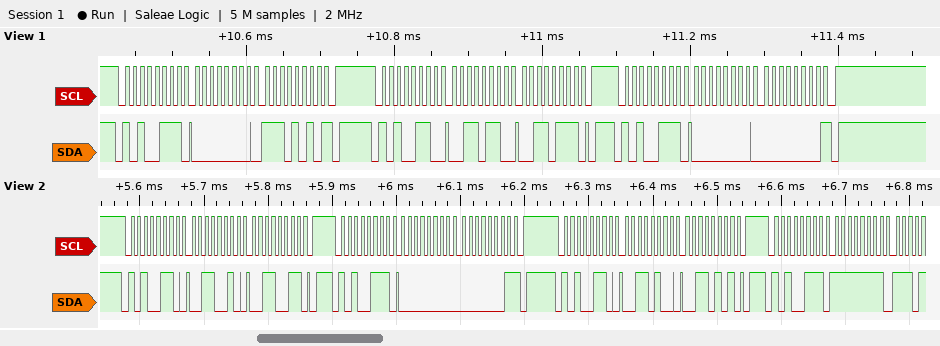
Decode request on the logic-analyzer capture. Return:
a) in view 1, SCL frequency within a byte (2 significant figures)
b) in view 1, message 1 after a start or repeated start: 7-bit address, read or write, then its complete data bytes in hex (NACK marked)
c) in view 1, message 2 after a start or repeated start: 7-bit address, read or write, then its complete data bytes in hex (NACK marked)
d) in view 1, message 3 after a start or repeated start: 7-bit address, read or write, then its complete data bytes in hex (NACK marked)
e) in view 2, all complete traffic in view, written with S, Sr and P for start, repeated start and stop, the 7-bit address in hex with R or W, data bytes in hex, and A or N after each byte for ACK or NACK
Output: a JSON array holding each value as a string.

["100 kHz", "0x53 read: 00 EA NACK", "0x53 write: 36 37", "0x53 read: 00 00 NACK", "S 53W A 32 A 33 A P S 53R A 00 A 01 N P S 53W A 34 A 35 A P S 53R A FF A"]
